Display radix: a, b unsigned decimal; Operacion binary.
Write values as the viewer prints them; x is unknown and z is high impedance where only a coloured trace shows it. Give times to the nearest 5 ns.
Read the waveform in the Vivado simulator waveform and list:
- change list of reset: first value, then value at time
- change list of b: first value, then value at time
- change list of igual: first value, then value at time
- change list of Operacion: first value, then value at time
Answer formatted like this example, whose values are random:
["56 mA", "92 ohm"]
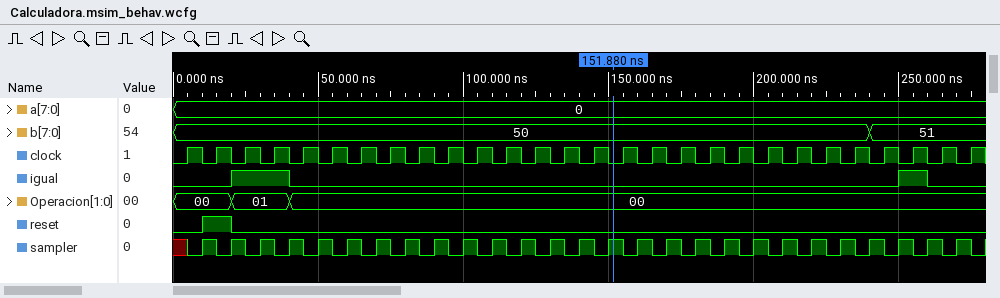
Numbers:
["0, 1 at 10 ns, 0 at 20 ns", "50, 51 at 240 ns", "0, 1 at 20 ns, 0 at 40 ns, 1 at 250 ns, 0 at 260 ns", "00, 01 at 20 ns, 00 at 40 ns"]
